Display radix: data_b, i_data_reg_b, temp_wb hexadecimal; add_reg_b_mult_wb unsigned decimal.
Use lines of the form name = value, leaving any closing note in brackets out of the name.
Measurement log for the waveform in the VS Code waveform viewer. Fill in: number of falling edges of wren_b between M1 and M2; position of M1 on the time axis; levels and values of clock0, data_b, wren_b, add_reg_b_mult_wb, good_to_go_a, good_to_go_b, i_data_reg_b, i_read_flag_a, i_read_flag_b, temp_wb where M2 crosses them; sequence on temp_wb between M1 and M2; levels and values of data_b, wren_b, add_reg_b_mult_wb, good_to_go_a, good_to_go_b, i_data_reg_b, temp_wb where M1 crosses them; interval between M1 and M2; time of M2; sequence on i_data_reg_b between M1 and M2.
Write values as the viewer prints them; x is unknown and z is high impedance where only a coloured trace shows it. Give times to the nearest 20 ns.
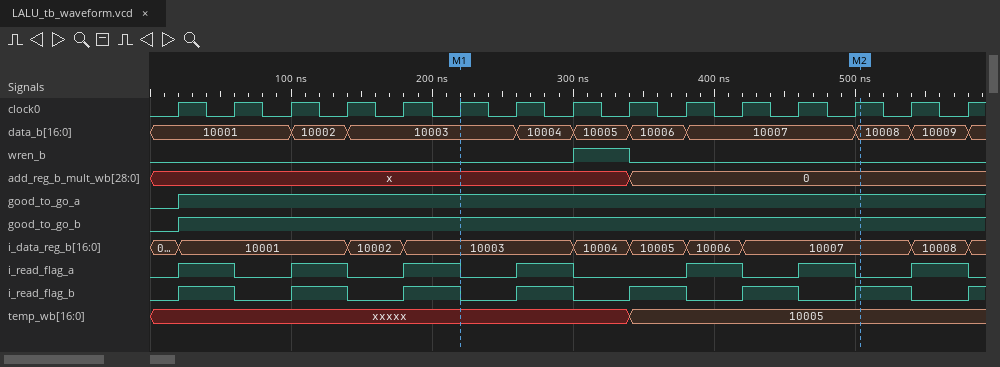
number of falling edges of wren_b between M1 and M2 = 1
position of M1 on the time axis = 220 ns
levels and values of clock0, data_b, wren_b, add_reg_b_mult_wb, good_to_go_a, good_to_go_b, i_data_reg_b, i_read_flag_a, i_read_flag_b, temp_wb where M2 crosses them = clock0=1, data_b=10008, wren_b=0, add_reg_b_mult_wb=0, good_to_go_a=1, good_to_go_b=1, i_data_reg_b=10007, i_read_flag_a=0, i_read_flag_b=1, temp_wb=10005
sequence on temp_wb between M1 and M2 = xxxxx, 10005
levels and values of data_b, wren_b, add_reg_b_mult_wb, good_to_go_a, good_to_go_b, i_data_reg_b, temp_wb where M1 crosses them = data_b=10003, wren_b=0, add_reg_b_mult_wb=x, good_to_go_a=1, good_to_go_b=1, i_data_reg_b=10003, temp_wb=xxxxx
interval between M1 and M2 = 280 ns
time of M2 = 500 ns
sequence on i_data_reg_b between M1 and M2 = 10003, 10004, 10005, 10006, 10007
